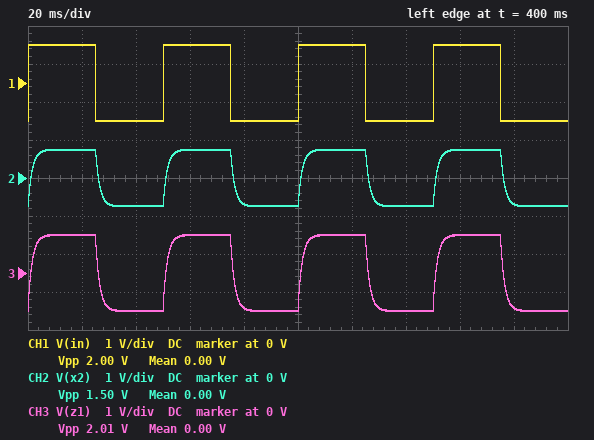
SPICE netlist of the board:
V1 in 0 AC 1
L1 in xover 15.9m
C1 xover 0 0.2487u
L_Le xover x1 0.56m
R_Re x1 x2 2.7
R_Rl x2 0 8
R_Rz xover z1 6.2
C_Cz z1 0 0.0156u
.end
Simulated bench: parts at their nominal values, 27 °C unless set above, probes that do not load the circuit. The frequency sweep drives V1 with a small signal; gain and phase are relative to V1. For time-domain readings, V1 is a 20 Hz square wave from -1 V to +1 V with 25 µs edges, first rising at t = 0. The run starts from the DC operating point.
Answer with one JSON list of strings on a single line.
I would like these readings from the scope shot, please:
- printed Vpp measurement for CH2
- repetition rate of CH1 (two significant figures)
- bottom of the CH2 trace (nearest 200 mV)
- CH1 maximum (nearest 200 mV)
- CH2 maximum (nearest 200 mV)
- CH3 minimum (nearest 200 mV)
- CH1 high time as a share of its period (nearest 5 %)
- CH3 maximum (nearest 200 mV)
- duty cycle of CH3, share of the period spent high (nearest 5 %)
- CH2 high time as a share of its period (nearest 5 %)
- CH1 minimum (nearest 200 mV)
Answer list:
["1.50 V", "20 Hz", "-800 mV", "1.0 V", "800 mV", "-1.0 V", "50 %", "1.0 V", "50 %", "50 %", "-1.0 V"]
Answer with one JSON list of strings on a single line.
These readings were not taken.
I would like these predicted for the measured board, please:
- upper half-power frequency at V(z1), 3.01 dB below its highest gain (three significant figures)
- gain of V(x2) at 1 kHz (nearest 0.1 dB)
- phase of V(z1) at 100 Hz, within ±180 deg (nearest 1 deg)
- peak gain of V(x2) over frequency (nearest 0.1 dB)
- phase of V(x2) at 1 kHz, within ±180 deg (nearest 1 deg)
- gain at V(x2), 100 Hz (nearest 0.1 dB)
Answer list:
["104 Hz", "-22.2 dB", "-42 deg", "-2.5 dB", "-85 deg", "-5.4 dB"]
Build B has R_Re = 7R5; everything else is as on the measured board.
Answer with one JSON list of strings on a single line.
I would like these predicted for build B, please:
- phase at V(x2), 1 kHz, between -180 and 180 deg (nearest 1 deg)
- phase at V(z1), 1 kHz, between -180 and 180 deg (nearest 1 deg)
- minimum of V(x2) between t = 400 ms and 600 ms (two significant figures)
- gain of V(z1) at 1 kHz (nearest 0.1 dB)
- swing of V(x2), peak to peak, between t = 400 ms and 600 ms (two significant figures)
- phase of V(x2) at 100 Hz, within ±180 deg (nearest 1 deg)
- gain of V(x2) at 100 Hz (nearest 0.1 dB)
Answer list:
["-83 deg", "-70 deg", "-520 mV", "-16.3 dB", "1.0 V", "-34 deg", "-7.3 dB"]
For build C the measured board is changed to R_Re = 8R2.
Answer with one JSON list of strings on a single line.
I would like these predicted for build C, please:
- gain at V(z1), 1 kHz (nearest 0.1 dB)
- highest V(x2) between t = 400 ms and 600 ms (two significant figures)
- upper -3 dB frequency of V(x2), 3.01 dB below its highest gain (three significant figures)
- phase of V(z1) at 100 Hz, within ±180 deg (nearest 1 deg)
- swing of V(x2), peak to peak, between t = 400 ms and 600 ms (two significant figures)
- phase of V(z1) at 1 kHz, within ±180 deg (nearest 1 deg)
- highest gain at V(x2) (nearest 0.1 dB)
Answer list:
["-15.9 dB", "490 mV", "157 Hz", "-31 deg", "990 mV", "-70 deg", "-6.1 dB"]
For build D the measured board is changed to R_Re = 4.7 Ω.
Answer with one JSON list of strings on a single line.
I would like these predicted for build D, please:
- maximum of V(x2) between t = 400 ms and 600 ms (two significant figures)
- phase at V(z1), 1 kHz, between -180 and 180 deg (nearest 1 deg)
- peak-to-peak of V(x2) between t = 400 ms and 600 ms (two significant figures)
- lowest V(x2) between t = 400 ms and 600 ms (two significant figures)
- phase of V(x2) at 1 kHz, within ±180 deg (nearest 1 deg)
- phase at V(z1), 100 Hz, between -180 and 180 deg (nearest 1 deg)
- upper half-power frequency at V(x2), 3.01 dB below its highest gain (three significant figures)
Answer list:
["630 mV", "-69 deg", "1.3 V", "-630 mV", "-84 deg", "-38 deg", "123 Hz"]
